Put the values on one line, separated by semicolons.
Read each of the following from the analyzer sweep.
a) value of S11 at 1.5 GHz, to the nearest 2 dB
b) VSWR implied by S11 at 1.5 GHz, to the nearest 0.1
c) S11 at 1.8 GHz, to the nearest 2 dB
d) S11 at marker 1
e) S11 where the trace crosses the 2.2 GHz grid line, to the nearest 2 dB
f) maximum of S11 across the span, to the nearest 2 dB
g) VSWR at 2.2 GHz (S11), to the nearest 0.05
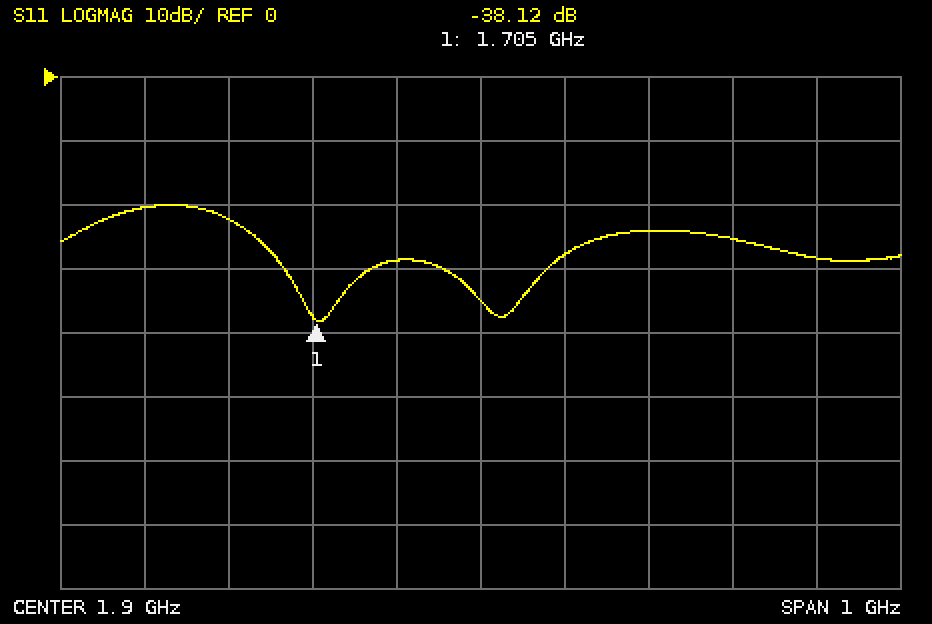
-20 dB; 1.2; -28 dB; -38.12 dB; -26 dB; -20 dB; 1.10
